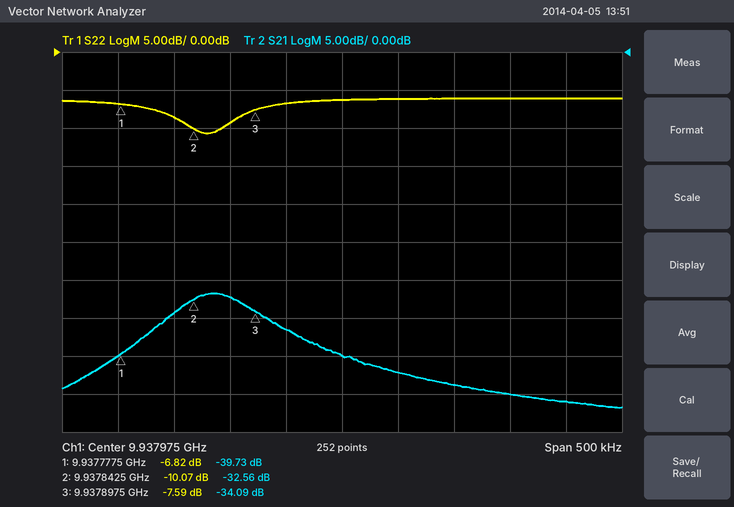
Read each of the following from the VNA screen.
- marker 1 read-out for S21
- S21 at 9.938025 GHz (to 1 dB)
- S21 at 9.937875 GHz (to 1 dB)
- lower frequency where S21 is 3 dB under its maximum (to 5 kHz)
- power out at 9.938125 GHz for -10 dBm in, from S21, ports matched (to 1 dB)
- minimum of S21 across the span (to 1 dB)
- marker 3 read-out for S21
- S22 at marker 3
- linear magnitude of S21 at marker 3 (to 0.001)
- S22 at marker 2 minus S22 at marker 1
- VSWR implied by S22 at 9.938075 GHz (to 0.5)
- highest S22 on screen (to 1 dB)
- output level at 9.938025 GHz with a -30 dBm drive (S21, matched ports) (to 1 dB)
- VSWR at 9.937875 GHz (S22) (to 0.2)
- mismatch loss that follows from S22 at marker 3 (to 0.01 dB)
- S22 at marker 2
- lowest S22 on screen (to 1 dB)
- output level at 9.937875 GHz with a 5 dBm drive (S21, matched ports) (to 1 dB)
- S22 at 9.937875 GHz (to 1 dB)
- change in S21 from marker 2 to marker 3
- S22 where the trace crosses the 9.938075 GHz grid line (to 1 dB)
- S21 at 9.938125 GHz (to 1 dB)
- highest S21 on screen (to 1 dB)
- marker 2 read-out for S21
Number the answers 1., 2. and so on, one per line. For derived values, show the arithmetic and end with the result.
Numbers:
1. -39.73 dB
2. -42 dB
3. -32 dB
4. 9.937820 GHz
5. -10 dBm + (-45 dB) = -55 dBm
6. -47 dB
7. -34.09 dB
8. -7.59 dB
9. 10^(-34.09/20) ≈ 0.020
10. -10.07 − (-6.82) = -3.25 dB
11. |Γ| = 10^(-6/20) = 0.5012; VSWR = (1 + 0.5012)/(1 − 0.5012) ≈ 3.0
12. -6 dB
13. -30 dBm + (-42 dB) = -72 dBm
14. |Γ| = 10^(-9/20) = 0.3548; VSWR = (1 + 0.3548)/(1 − 0.3548) ≈ 2.10, so 2.0 to the nearest 0.2
15. −10 log10(1 − 10^(-7.59/10)) ≈ 0.83 dB
16. -10.07 dB
17. -11 dB
18. 5 dBm + (-32 dB) = -27 dBm
19. -9 dB
20. -34.09 − (-32.56) = -1.53 dB
21. -6 dB
22. -45 dB
23. -32 dB
24. -32.56 dB
